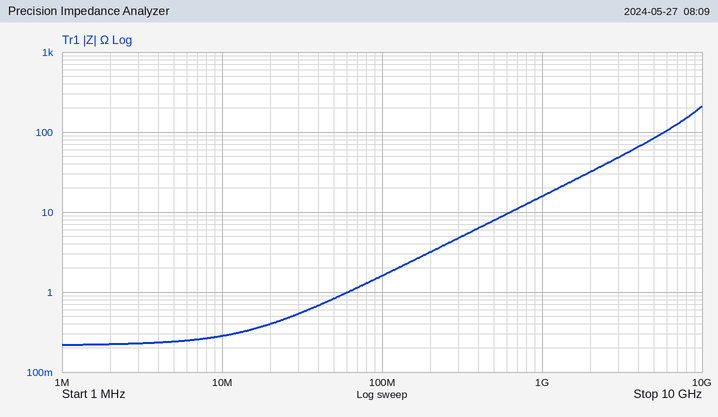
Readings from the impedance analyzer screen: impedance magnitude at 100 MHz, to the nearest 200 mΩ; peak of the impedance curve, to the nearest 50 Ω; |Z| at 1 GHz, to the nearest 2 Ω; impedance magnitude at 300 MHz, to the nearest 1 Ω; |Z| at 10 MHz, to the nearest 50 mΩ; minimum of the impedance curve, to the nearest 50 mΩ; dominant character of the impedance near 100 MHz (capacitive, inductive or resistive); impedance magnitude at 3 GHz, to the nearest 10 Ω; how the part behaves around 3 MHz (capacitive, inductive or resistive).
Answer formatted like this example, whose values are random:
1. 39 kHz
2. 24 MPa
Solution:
1. 1.6 Ω
2. 200 Ω
3. 16 Ω
4. 5 Ω
5. 300 mΩ
6. 200 mΩ
7. inductive
8. 50 Ω
9. resistive
